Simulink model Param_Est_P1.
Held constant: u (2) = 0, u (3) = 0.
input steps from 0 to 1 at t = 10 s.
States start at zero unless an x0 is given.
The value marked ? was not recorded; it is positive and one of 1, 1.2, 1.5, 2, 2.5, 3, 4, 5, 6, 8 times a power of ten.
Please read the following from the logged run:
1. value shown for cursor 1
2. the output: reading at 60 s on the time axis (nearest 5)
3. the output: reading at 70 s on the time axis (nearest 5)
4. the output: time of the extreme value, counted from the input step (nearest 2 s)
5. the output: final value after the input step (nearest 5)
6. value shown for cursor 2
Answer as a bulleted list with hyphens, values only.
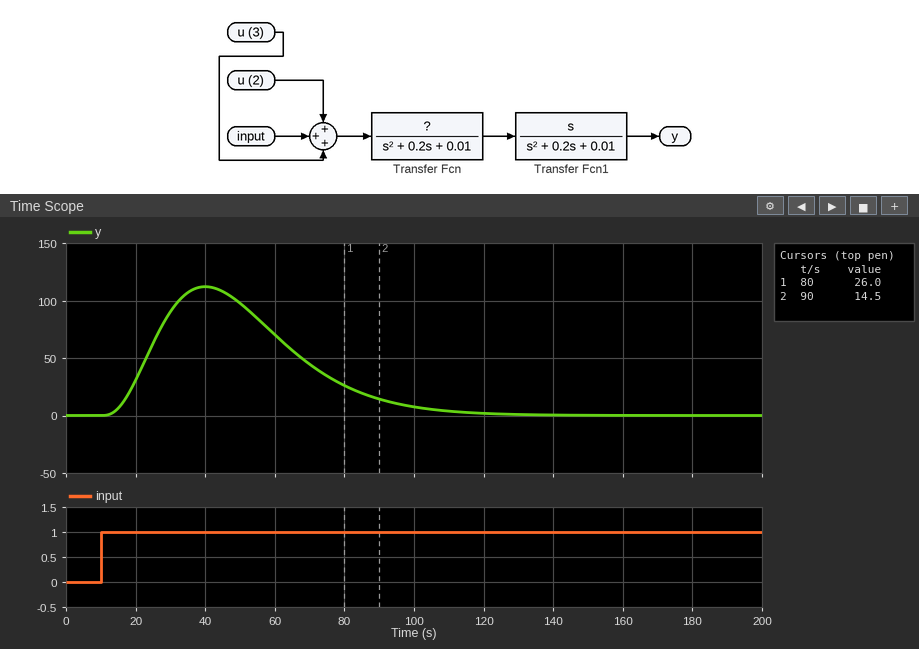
- 26.0
- 70
- 45
- 30 s
- 0
- 14.5
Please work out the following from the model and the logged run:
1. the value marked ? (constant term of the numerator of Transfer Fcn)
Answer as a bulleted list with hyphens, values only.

- 0.5
